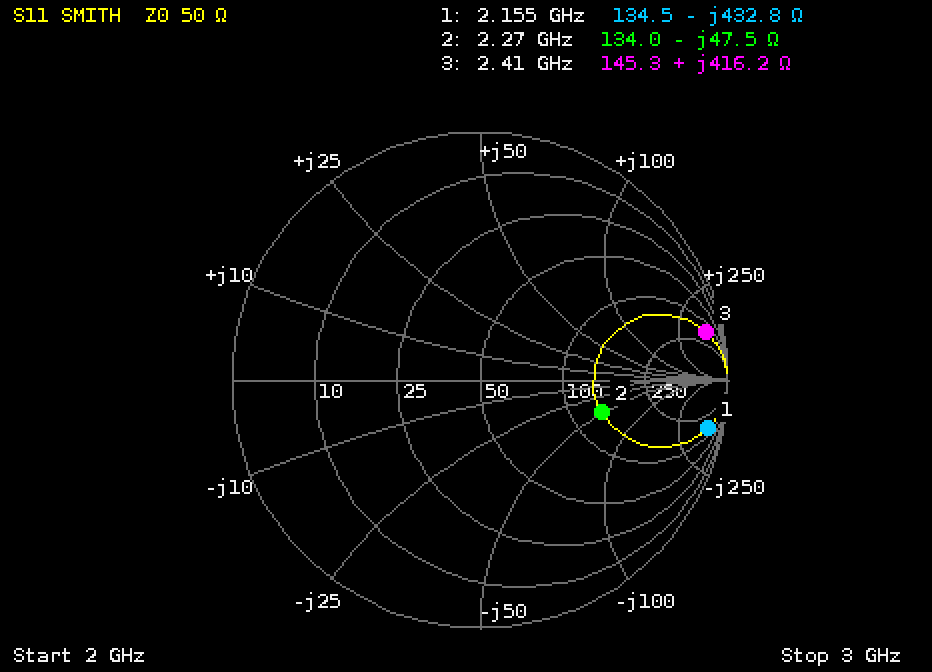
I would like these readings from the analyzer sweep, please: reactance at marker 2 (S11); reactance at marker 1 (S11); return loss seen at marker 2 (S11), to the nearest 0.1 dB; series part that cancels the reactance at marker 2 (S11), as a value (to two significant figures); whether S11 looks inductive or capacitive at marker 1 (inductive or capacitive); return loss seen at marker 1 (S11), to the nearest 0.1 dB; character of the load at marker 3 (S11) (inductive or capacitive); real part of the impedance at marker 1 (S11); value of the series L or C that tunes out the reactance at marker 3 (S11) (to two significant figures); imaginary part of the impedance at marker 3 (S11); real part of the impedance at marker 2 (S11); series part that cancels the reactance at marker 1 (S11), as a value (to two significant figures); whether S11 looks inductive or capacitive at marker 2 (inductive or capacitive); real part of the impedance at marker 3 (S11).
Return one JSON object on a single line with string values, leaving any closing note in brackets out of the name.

{"reactance at marker 2": "-47.5 Ω", "reactance at marker 1": "-432.8 Ω", "return loss seen at marker 2 (S11), to the nearest 0.1 dB": "5.9 dB", "series part that cancels the reactance at marker 2 (S11), as a value": "3.3 nH", "whether S11 looks inductive or capacitive at marker 1": "capacitive", "return loss seen at marker 1 (S11), to the nearest 0.1 dB": "0.6 dB", "character of the load at marker 3 (S11)": "inductive", "real part of the impedance at marker 1": "134.5 Ω", "value of the series L or C that tunes out the reactance at marker 3 (S11)": "160 fF", "imaginary part of the impedance at marker 3": "+416.2 Ω", "real part of the impedance at marker 2": "134.0 Ω", "series part that cancels the reactance at marker 1 (S11), as a value": "32 nH", "whether S11 looks inductive or capacitive at marker 2": "capacitive", "real part of the impedance at marker 3": "145.3 Ω"}
